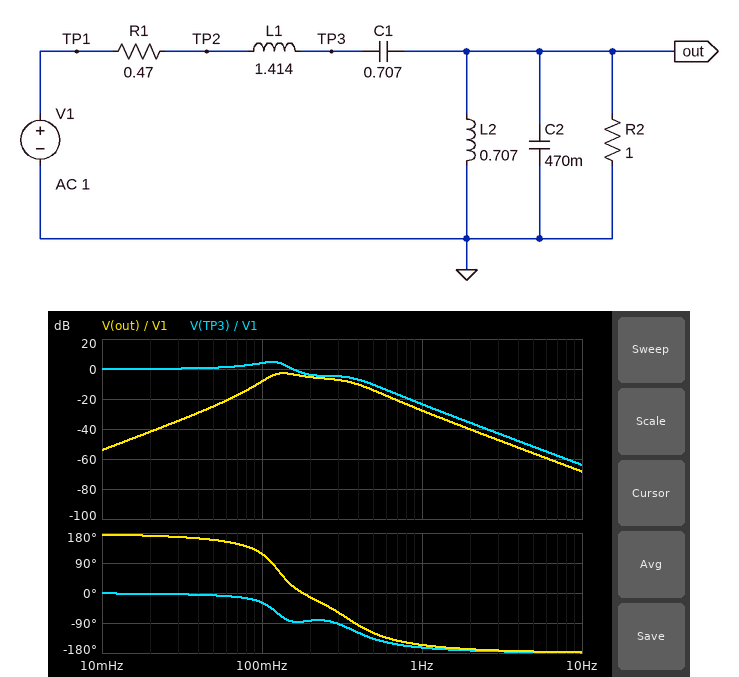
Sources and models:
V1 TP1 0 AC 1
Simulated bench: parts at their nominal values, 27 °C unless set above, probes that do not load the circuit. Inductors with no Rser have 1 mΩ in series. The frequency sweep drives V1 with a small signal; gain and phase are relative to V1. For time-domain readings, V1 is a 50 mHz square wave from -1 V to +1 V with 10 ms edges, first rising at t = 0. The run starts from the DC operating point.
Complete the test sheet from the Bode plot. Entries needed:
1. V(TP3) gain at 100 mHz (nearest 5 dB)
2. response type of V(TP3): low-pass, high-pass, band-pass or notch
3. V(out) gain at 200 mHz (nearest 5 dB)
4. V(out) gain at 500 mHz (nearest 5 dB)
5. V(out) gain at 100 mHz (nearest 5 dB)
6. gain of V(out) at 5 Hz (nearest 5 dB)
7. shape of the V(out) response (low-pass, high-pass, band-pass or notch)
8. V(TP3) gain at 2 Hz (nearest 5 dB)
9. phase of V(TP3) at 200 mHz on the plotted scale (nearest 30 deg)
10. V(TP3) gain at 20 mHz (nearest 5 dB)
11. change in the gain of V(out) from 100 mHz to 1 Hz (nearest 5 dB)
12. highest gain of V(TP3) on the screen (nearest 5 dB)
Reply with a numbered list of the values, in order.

1. 5 dB
2. low-pass
3. -5 dB
4. -15 dB
5. -10 dB
6. -55 dB
7. band-pass
8. -35 dB
9. -90 deg
10. 0 dB
11. -20 dB
12. 5 dB
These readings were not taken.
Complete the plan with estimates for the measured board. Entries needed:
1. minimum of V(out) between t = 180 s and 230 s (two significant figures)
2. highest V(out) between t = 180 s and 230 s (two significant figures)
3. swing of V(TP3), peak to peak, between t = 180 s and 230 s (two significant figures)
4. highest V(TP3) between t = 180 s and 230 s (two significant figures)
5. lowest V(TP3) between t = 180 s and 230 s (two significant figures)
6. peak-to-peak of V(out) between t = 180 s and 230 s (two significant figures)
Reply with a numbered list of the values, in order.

1. -520 mV
2. 520 mV
3. 3.1 V
4. 1.5 V
5. -1.5 V
6. 1.0 V
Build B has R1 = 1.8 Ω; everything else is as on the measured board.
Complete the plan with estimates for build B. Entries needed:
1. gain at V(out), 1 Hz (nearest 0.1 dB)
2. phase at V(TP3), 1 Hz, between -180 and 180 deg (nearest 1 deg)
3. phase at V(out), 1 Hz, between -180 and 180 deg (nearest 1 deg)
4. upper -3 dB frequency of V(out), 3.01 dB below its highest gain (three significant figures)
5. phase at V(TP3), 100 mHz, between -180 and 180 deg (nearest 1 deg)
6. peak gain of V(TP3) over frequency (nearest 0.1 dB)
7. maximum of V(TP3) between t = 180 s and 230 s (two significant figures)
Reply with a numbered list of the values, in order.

1. -27.9 dB
2. -155 deg
3. -147 deg
4. 418 mHz
5. -58 deg
6. 0.1 dB
7. 1.1 V
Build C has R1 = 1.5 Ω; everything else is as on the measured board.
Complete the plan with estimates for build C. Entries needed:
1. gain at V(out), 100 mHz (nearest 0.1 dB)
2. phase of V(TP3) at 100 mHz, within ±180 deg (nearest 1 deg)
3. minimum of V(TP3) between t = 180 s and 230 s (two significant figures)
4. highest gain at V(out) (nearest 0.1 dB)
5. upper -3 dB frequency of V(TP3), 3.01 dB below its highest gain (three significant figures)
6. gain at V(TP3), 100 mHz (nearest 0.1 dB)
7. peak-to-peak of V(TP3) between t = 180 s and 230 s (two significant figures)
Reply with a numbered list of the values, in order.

1. -12.7 dB
2. -54 deg
3. -1.2 V
4. -9.1 dB
5. 126 mHz
6. -0.5 dB
7. 2.4 V
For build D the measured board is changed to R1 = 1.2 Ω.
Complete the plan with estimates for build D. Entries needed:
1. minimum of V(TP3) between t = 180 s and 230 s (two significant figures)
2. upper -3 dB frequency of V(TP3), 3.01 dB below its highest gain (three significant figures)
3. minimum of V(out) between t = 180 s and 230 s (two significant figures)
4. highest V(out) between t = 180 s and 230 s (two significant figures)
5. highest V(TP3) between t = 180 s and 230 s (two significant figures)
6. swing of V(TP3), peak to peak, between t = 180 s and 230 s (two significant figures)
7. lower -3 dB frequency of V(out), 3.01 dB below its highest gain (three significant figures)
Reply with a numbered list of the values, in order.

1. -1.3 V
2. 134 mHz
3. -380 mV
4. 380 mV
5. 1.3 V
6. 2.5 V
7. 104 mHz
